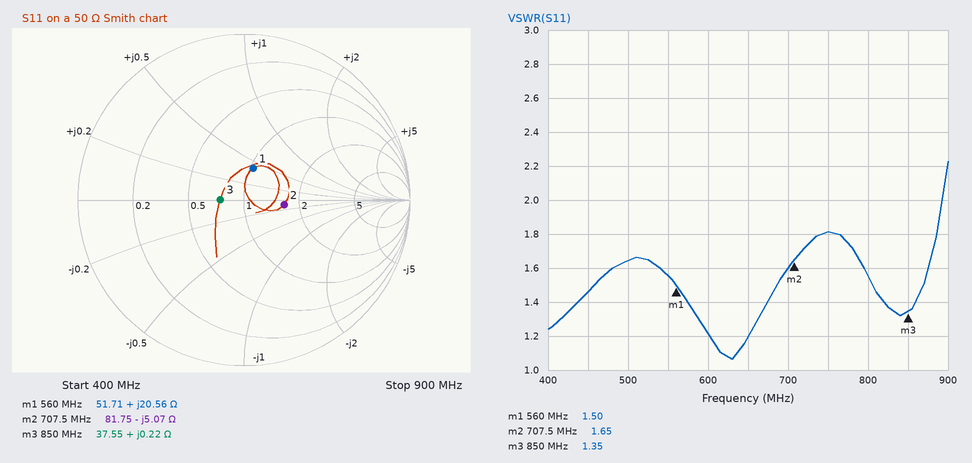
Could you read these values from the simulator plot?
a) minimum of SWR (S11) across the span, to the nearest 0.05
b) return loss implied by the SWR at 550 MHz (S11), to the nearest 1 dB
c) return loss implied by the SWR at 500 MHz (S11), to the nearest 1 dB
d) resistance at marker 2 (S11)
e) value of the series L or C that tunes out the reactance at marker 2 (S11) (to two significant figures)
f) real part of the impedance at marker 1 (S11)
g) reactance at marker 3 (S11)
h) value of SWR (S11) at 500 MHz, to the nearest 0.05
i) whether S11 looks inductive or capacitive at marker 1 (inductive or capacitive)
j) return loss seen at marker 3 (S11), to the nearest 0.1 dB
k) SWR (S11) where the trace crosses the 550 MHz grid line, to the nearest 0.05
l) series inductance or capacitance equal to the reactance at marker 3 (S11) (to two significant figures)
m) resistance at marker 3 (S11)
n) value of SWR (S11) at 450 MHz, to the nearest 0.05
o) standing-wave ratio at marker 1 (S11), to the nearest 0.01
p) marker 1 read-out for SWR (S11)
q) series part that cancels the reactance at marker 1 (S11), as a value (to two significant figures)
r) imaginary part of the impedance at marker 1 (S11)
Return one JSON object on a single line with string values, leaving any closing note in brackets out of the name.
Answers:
{"minimum of SWR (S11) across the span, to the nearest 0.05": "1.05", "return loss implied by the SWR at 550 MHz (S11), to the nearest 1 dB": "13 dB", "return loss implied by the SWR at 500 MHz (S11), to the nearest 1 dB": "12 dB", "resistance at marker 2": "81.75 Ω", "value of the series L or C that tunes out the reactance at marker 2 (S11)": "1.1 nH", "real part of the impedance at marker 1": "51.71 Ω", "reactance at marker 3": "+0.22 Ω", "value of SWR (S11) at 500 MHz, to the nearest 0.05": "1.65", "whether S11 looks inductive or capacitive at marker 1": "inductive", "return loss seen at marker 3 (S11), to the nearest 0.1 dB": "16.9 dB", "SWR (S11) where the trace crosses the 550 MHz grid line, to the nearest 0.05": "1.55", "series inductance or capacitance equal to the reactance at marker 3 (S11)": "41 pH", "resistance at marker 3": "37.55 Ω", "value of SWR (S11) at 450 MHz, to the nearest 0.05": "1.45", "standing-wave ratio at marker 1 (S11), to the nearest 0.01": "1.50", "marker 1 read-out for SWR": "1.50", "series part that cancels the reactance at marker 1 (S11), as a value": "14 pF", "imaginary part of the impedance at marker 1": "+20.56 Ω"}
